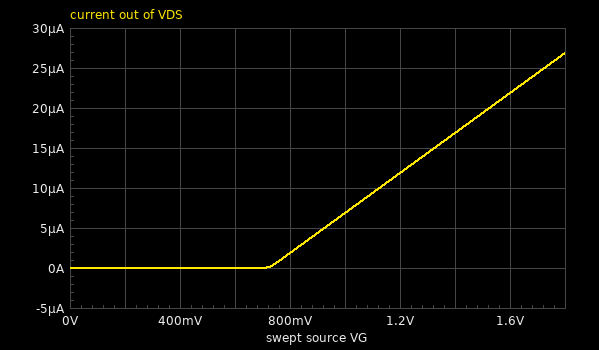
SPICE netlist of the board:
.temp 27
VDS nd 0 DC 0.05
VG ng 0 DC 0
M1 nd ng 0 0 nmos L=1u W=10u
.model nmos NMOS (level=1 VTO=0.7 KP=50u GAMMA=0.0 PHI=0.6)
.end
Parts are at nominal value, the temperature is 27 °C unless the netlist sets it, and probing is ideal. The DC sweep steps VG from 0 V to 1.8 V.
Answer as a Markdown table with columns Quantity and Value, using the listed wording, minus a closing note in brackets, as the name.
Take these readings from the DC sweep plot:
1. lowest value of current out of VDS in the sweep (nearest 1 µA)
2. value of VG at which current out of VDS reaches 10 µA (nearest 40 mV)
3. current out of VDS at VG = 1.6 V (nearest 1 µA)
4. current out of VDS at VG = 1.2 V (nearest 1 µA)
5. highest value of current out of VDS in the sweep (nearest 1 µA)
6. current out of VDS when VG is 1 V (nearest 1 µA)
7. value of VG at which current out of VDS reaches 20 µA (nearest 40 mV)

| Quantity | Value |
|---|---|
| lowest value of current out of VDS in the sweep | 0 A |
| value of VG at which current out of VDS reaches 10 µA | 1.12 V |
| current out of VDS at VG = 1.6 V | 22 µA |
| current out of VDS at VG = 1.2 V | 12 µA |
| highest value of current out of VDS in the sweep | 27 µA |
| current out of VDS when VG is 1 V | 7 µA |
| value of VG at which current out of VDS reaches 20 µA | 1.52 V |
